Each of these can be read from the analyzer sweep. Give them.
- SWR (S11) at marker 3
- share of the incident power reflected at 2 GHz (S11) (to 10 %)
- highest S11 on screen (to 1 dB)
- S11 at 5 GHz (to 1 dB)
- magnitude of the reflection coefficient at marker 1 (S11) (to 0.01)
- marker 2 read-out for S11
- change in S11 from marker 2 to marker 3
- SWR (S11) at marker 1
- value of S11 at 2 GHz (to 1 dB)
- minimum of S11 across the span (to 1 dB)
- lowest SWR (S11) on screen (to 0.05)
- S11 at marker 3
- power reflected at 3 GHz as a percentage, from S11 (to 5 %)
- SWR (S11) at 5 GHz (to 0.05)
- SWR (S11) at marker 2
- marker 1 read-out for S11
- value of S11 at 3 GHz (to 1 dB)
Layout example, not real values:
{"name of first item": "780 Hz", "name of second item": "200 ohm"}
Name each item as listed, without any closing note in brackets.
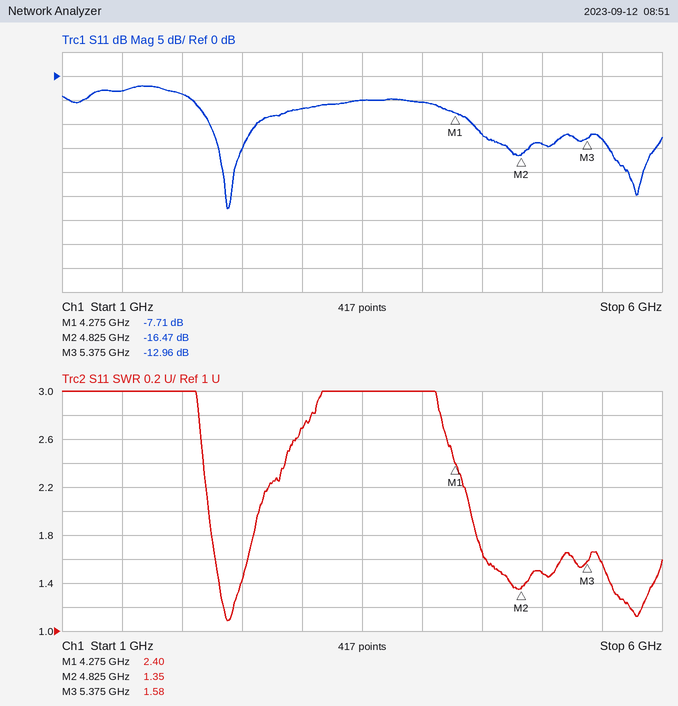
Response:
{"SWR (S11) at marker 3": "1.58", "share of the incident power reflected at 2 GHz (S11)": "40 %", "highest S11 on screen": "-2 dB", "S11 at 5 GHz": "-14 dB", "magnitude of the reflection coefficient at marker 1 (S11)": "0.41", "marker 2 read-out for S11": "-16.47 dB", "change in S11 from marker 2 to marker 3": "3.51 dB", "SWR (S11) at marker 1": "2.40", "value of S11 at 2 GHz": "-4 dB", "minimum of S11 across the span": "-28 dB", "lowest SWR (S11) on screen": "1.10", "S11 at marker 3": "-12.96 dB", "power reflected at 3 GHz as a percentage, from S11": "20 %", "SWR (S11) at 5 GHz": "1.50", "SWR (S11) at marker 2": "1.35", "marker 1 read-out for S11": "-7.71 dB", "value of S11 at 3 GHz": "-7 dB"}
